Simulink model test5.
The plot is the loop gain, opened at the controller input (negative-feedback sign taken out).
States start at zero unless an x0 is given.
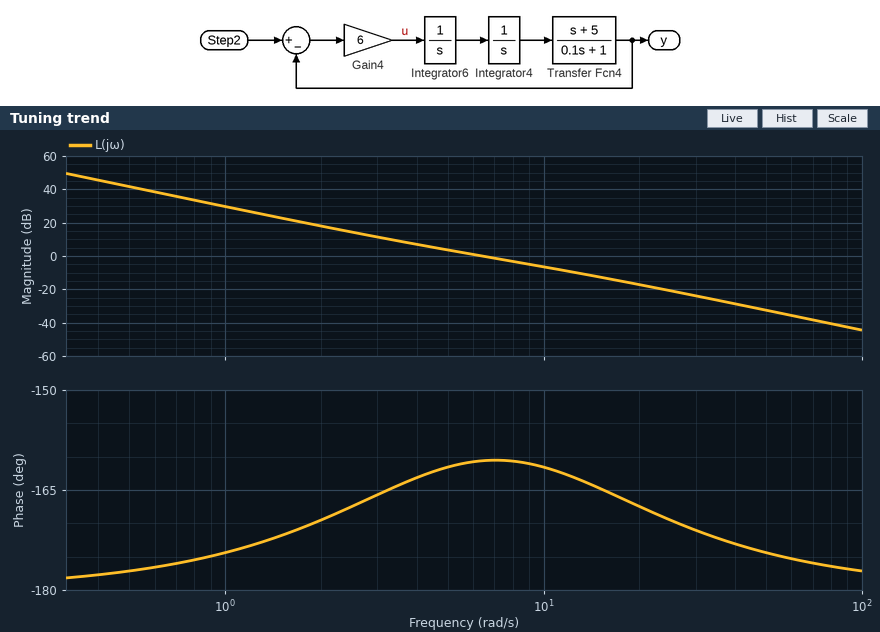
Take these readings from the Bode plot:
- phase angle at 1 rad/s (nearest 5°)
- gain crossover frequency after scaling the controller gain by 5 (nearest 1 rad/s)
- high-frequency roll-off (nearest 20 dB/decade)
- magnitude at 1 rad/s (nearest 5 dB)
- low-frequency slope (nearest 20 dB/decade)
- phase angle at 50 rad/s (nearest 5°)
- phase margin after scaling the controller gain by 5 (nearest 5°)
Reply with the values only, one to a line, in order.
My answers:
-175°
16 rad/s
-40 dB/decade
30 dB
-40 dB/decade
-175°
15°
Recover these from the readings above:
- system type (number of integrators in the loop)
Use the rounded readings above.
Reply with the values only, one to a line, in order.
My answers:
2
